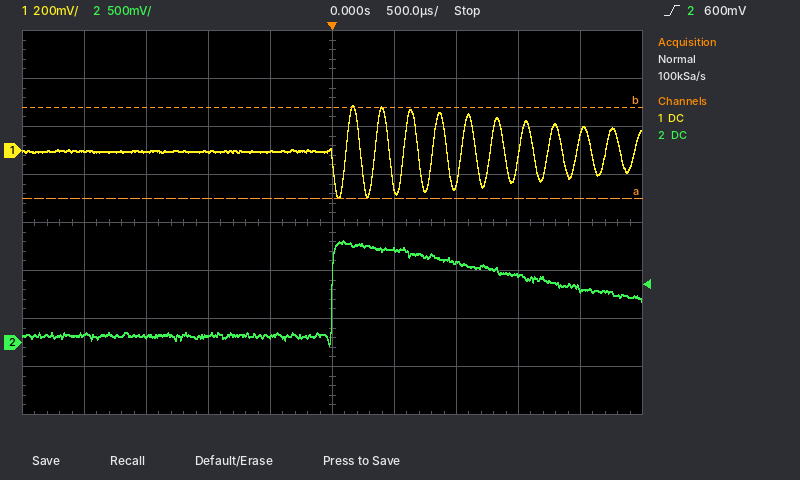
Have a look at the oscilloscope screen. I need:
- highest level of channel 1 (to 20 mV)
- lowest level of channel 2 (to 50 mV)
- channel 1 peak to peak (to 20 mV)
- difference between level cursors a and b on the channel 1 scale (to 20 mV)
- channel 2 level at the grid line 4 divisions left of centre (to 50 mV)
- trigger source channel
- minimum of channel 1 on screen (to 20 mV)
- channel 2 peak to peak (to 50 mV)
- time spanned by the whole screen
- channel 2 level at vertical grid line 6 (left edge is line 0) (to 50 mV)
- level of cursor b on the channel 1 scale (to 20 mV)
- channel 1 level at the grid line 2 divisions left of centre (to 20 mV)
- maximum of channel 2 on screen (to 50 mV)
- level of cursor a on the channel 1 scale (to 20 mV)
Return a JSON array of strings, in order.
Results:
["180 mV", "-50 mV", "380 mV", "380 mV", "100 mV", "channel 2", "-200 mV", "1.10 V", "5 ms", "950 mV", "180 mV", "0 mV", "1.05 V", "-200 mV"]
